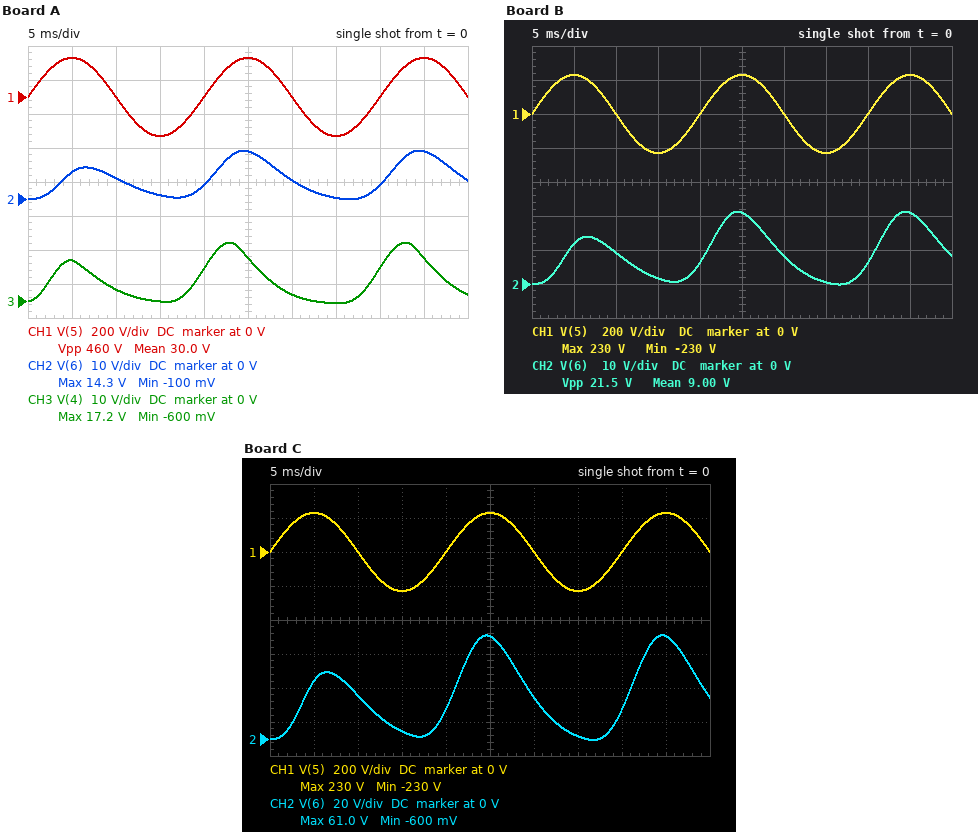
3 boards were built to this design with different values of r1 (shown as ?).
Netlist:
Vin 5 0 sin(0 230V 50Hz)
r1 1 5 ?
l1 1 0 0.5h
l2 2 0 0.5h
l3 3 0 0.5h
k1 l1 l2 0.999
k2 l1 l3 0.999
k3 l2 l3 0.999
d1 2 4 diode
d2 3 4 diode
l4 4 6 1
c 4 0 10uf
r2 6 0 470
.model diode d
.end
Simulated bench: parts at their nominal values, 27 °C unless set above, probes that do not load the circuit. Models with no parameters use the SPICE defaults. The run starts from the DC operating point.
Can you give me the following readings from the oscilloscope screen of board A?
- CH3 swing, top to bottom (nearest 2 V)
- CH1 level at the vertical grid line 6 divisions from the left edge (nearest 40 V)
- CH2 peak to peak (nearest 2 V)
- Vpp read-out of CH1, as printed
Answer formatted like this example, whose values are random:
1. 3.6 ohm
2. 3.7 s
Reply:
1. 18 V
2. 0 V
3. 14 V
4. 460 V
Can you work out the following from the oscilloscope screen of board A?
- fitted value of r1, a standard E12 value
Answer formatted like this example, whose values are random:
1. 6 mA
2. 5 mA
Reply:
1. 2.7 kΩ
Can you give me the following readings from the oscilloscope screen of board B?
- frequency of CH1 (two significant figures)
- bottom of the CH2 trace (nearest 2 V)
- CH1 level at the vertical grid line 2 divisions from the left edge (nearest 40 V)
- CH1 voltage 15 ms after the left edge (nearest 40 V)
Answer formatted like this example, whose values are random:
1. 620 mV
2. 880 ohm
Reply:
1. 50 Hz
2. 0 V
3. 0 V
4. -240 V
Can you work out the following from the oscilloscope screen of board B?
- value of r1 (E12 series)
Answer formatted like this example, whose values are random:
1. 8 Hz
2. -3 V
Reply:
1. 1.8 kΩ
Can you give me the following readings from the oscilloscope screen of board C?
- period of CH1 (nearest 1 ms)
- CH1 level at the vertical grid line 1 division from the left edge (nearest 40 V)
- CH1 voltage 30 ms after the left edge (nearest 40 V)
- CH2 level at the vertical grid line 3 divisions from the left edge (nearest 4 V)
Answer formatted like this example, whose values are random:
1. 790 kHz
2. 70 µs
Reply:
1. 20 ms
2. 240 V
3. 0 V
4. 4 V
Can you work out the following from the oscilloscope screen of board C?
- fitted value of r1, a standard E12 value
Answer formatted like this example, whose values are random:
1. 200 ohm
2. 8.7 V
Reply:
1. 560 Ω
